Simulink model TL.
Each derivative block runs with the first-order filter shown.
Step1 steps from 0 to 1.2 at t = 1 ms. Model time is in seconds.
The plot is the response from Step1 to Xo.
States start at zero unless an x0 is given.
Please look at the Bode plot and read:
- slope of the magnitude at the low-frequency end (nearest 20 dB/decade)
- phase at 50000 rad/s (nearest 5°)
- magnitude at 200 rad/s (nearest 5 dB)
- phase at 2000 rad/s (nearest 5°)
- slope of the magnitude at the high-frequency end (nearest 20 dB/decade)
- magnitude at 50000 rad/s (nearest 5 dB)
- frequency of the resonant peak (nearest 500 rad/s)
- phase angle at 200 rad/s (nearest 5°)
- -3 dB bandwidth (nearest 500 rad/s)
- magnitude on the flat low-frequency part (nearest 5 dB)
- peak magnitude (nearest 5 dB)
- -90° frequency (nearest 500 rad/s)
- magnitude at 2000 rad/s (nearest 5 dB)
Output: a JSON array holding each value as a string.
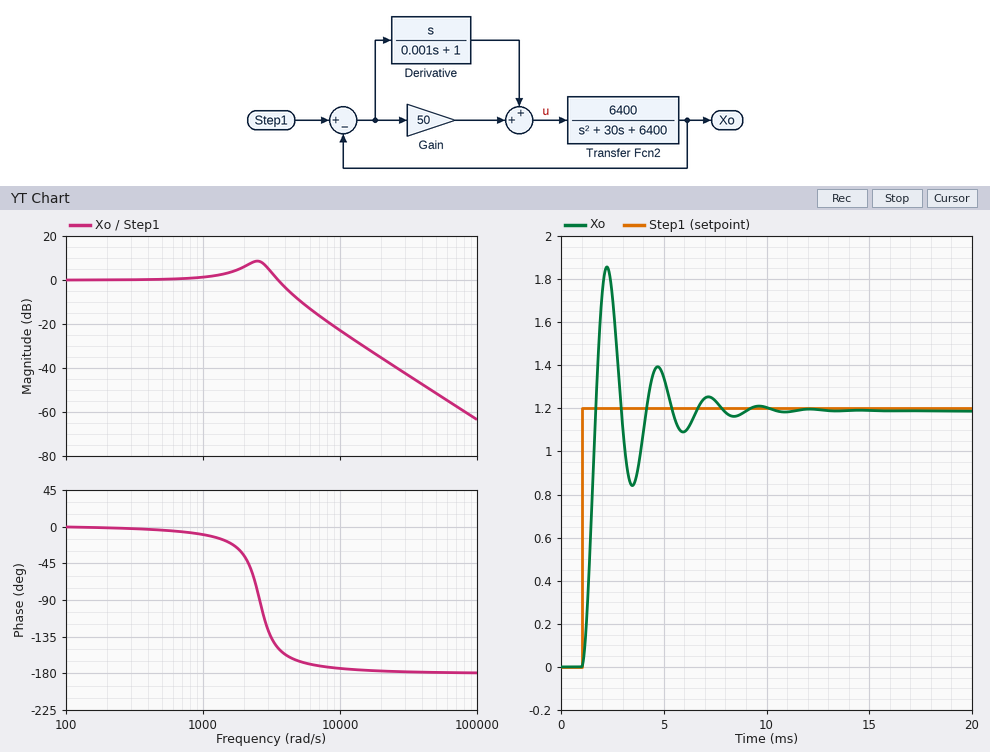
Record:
["0 dB/decade", "-180°", "0 dB", "-35°", "-40 dB/decade", "-50 dB", "2500 rad/s", "0°", "4000 rad/s", "0 dB", "10 dB", "2500 rad/s", "5 dB"]
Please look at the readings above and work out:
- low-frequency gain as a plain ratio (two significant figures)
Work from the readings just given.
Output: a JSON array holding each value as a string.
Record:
["1.0"]
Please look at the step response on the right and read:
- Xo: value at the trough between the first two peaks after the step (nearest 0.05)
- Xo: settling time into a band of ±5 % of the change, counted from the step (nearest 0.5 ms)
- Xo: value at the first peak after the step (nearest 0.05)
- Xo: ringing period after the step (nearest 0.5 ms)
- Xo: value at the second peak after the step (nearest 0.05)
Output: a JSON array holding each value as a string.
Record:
["0.85", "6.5 ms", "1.85", "2.5 ms", "1.40"]
